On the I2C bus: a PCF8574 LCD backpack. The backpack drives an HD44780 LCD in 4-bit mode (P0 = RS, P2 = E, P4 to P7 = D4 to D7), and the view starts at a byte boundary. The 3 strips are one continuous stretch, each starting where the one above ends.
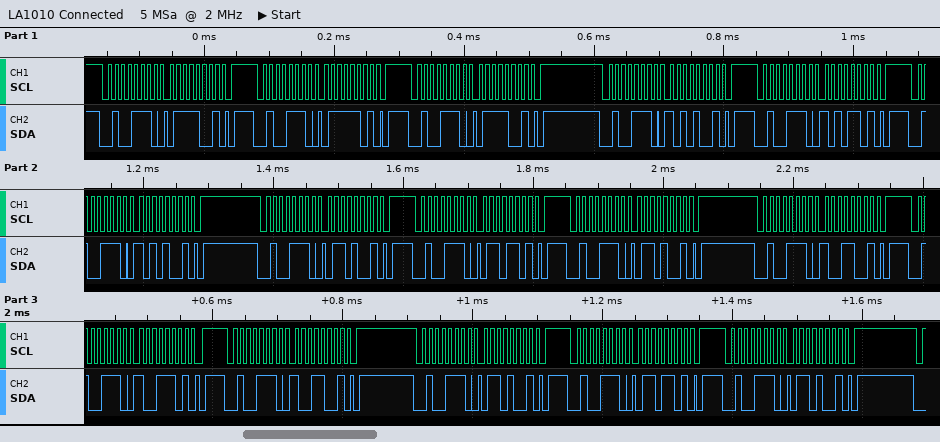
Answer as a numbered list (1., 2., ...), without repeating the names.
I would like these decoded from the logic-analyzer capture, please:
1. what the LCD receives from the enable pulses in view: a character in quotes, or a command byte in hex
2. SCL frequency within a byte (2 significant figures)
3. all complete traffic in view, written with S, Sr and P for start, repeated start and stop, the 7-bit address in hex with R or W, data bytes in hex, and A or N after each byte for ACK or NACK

1. 'z' 'i'
2. 100 kHz
3. S 27W A 79 A P S 27W A 7D A P S 27W A 79 A P S 27W A A9 A P S 27W A AD A P S 27W A A9 A P S 27W A 69 A P S 27W A 6D A P S 27W A 69 A P S 27W A 99 A P S 27W A 9D A P S 27W A 99 A P S 27W A 69 A P S 27W A 6D A P S 27W A 69 A P
